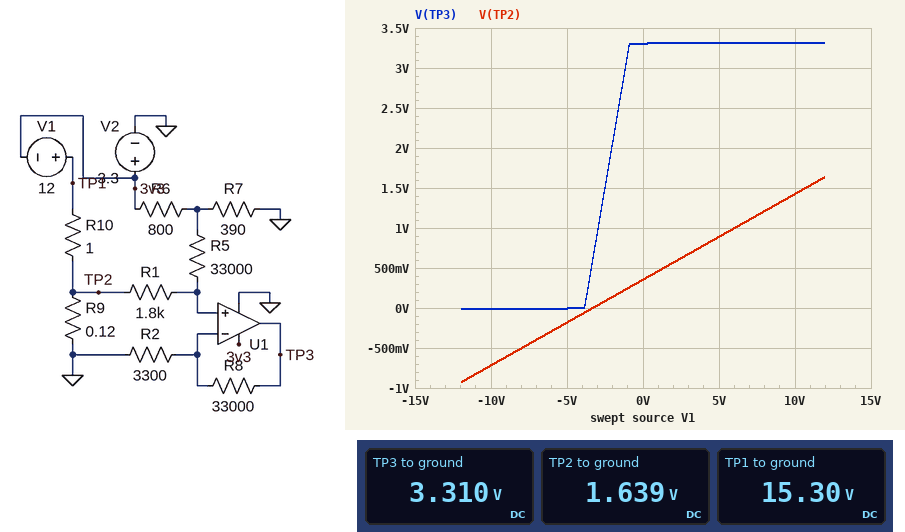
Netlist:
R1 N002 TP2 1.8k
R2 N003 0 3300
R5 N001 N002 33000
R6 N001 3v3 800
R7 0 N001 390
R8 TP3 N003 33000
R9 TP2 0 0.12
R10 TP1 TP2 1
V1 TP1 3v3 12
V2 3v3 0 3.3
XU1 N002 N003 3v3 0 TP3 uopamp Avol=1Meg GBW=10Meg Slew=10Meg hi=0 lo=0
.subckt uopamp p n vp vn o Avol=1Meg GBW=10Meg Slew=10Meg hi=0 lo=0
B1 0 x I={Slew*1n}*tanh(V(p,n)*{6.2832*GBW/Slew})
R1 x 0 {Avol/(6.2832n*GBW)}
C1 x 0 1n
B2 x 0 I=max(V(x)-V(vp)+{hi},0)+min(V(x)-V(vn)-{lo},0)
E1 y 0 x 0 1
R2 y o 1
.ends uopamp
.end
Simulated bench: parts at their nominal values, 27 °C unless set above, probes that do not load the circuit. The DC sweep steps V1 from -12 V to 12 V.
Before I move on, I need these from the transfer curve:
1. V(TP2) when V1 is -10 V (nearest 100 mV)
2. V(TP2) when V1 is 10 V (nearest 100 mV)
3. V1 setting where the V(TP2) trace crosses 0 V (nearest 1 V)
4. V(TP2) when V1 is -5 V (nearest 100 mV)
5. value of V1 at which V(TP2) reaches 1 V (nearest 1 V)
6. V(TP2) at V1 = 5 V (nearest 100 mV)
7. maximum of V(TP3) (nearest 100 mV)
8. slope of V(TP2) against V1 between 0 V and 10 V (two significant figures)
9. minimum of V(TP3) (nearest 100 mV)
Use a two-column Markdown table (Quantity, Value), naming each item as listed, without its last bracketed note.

| Quantity | Value |
|---|---|
| V(TP2) when V1 is -10 V | -700 mV |
| V(TP2) when V1 is 10 V | 1.4 V |
| V1 setting where the V(TP2) trace crosses 0 V | -3 V |
| V(TP2) when V1 is -5 V | -200 mV |
| value of V1 at which V(TP2) reaches 1 V | 6 V |
| V(TP2) at V1 = 5 V | 900 mV |
| maximum of V(TP3) | 3.3 V |
| slope of V(TP2) against V1 between 0 V and 10 V | 0.11 V/V |
| minimum of V(TP3) | 0 V |
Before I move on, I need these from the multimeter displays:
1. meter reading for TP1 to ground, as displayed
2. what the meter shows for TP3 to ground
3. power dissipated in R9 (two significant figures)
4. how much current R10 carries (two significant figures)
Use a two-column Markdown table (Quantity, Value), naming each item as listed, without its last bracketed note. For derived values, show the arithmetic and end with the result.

| Quantity | Value |
|---|---|
| meter reading for TP1 to ground, as displayed | 15.30 V |
| what the meter shows for TP3 to ground | 3.310 V |
| power dissipated in R9 | (1.639 V)^2 / 120 mΩ = 22 W |
| how much current R10 carries | (15.3 V - 1.639 V) / 1 Ω = 14 A |
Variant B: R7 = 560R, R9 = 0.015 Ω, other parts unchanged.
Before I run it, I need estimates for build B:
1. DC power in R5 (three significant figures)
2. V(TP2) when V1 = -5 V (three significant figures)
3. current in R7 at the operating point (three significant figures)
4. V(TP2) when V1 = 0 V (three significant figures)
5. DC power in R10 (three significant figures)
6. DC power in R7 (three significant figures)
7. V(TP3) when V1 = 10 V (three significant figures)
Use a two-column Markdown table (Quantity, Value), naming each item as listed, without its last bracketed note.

| Quantity | Value |
|---|---|
| DC power in R5 | 34.3 µW |
| V(TP2) when V1 = -5 V | -25.1 mV |
| current in R7 at the operating point | 2.41 mA |
| V(TP2) when V1 = 0 V | 48.8 mV |
| DC power in R10 | 227 W |
| DC power in R7 | 3.25 mW |
| V(TP3) when V1 = 10 V | 2.82 V |
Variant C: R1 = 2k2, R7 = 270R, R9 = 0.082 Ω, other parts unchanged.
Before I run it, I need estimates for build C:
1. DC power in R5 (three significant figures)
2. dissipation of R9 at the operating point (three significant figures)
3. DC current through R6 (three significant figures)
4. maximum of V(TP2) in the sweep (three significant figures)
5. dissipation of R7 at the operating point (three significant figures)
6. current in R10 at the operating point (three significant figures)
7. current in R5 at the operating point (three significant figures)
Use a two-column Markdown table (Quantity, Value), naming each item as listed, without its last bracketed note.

| Quantity | Value |
|---|---|
| DC power in R5 | 2.81 µW |
| dissipation of R9 at the operating point | 16.4 W |
| DC current through R6 | 3.08 mA |
| maximum of V(TP2) in the sweep | 1.16 V |
| dissipation of R7 at the operating point | 2.58 mW |
| current in R10 at the operating point | 14.1 A |
| current in R5 at the operating point | 9.23 µA |
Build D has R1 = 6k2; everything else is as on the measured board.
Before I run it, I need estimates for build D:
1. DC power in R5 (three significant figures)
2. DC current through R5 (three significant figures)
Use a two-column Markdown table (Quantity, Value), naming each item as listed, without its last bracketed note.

| Quantity | Value |
|---|---|
| DC power in R5 | 6.59 µW |
| DC current through R5 | 14.1 µA |
